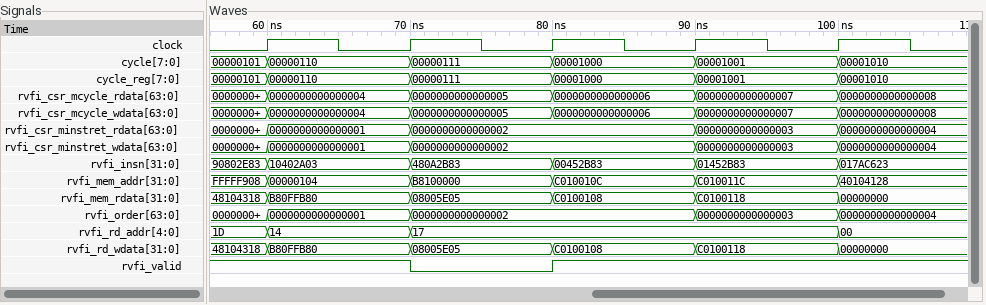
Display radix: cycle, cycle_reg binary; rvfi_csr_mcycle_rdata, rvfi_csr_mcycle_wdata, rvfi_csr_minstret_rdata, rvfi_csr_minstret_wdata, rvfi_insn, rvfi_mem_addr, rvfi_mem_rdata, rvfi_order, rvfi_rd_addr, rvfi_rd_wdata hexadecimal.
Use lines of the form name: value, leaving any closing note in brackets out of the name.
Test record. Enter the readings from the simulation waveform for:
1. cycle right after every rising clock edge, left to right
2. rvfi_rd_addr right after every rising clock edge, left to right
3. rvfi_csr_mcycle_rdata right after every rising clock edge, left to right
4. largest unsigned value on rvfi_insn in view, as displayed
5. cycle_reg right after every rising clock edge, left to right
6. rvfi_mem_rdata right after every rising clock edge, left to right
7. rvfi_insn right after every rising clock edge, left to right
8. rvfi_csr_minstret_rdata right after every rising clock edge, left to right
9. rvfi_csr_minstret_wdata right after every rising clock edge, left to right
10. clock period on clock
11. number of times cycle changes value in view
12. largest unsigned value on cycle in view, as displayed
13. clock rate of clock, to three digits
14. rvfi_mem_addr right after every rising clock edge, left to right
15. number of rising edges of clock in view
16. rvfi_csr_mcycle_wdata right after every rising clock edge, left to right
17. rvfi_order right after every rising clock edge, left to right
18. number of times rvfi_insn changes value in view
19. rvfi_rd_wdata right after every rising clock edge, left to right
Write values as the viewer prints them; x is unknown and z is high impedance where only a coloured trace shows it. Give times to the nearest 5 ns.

cycle right after every rising clock edge, left to right: 00000110, 00000111, 00001000, 00001001, 00001010
rvfi_rd_addr right after every rising clock edge, left to right: 14, 17, 17, 17, 00
rvfi_csr_mcycle_rdata right after every rising clock edge, left to right: 0000000000000004, 0000000000000005, 0000000000000006, 0000000000000007, 0000000000000008
largest unsigned value on rvfi_insn in view, as displayed: 90802E83
cycle_reg right after every rising clock edge, left to right: 00000110, 00000111, 00001000, 00001001, 00001010
rvfi_mem_rdata right after every rising clock edge, left to right: B80FFB80, 08005E05, C0100108, C0100118, 00000000
rvfi_insn right after every rising clock edge, left to right: 10402A03, 480A2B83, 00452B83, 01452B83, 017AC623
rvfi_csr_minstret_rdata right after every rising clock edge, left to right: 0000000000000001, 0000000000000002, 0000000000000002, 0000000000000003, 0000000000000004
rvfi_csr_minstret_wdata right after every rising clock edge, left to right: 0000000000000001, 0000000000000002, 0000000000000002, 0000000000000003, 0000000000000004
clock period on clock: 10 ns
number of times cycle changes value in view: 5
largest unsigned value on cycle in view, as displayed: 00001010
clock rate of clock, to three digits: 100 MHz
rvfi_mem_addr right after every rising clock edge, left to right: 00000104, B8100000, C010010C, C010011C, 40104128
number of rising edges of clock in view: 5
rvfi_csr_mcycle_wdata right after every rising clock edge, left to right: 0000000000000004, 0000000000000005, 0000000000000006, 0000000000000007, 0000000000000008
rvfi_order right after every rising clock edge, left to right: 0000000000000001, 0000000000000002, 0000000000000002, 0000000000000003, 0000000000000004
number of times rvfi_insn changes value in view: 5
rvfi_rd_wdata right after every rising clock edge, left to right: B80FFB80, 08005E05, C0100108, C0100118, 00000000
